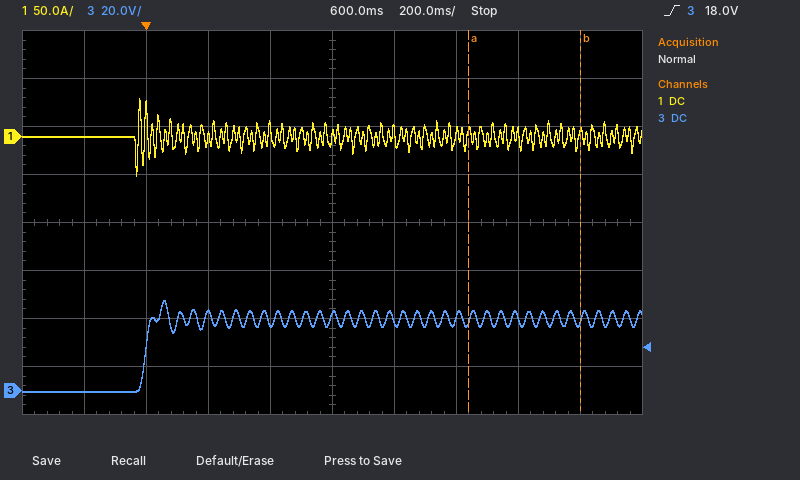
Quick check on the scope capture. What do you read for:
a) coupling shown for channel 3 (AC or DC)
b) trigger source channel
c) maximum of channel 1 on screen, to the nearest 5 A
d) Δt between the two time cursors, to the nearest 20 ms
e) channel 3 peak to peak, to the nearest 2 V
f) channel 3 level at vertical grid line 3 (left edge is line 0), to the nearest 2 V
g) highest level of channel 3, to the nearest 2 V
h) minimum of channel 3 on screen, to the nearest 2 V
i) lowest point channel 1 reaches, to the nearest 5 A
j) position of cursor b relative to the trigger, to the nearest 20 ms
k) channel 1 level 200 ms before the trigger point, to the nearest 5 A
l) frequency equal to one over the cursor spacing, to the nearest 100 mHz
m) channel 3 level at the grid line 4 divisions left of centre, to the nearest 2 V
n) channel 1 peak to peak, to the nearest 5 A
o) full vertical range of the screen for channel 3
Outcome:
DC
channel 3
40 A
360 ms
38 V
32 V
38 V
0 V
-40 A
+1.40 s
0 A
2.8 Hz
0 V
80 A
160 V
